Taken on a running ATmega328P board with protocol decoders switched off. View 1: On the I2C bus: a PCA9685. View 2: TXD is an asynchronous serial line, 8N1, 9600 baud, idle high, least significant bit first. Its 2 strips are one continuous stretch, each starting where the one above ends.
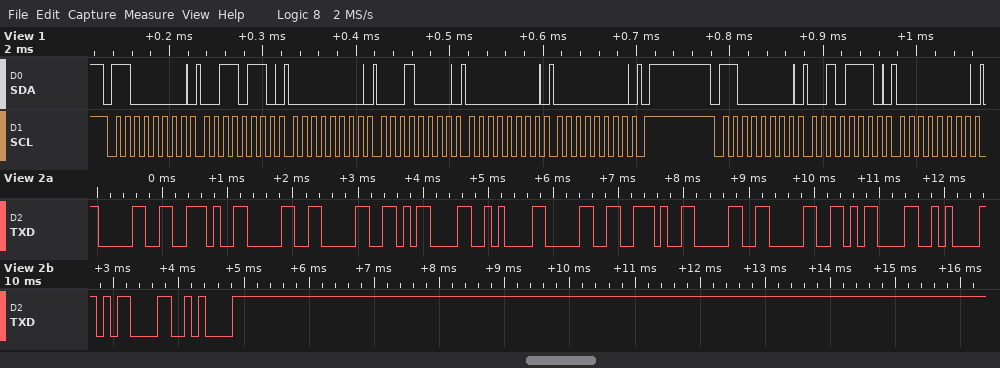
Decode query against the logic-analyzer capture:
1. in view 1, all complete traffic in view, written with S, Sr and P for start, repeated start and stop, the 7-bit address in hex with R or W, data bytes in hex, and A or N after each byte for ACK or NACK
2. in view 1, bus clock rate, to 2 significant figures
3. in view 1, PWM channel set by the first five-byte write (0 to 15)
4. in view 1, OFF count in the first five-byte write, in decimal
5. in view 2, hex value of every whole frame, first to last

S 60W A 36 A 00 A 10 A 00 A 00 A P S 60W A 2E A 00 A
100 kHz
12
0
30 2E 30 30 0D 0A 30 2E 30 30 0D 0A 0D 0A
